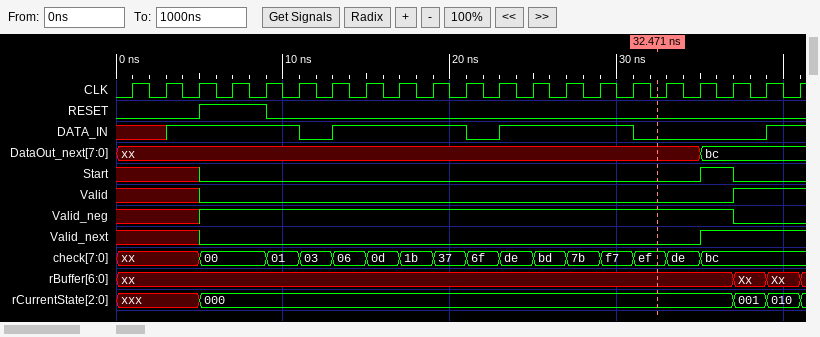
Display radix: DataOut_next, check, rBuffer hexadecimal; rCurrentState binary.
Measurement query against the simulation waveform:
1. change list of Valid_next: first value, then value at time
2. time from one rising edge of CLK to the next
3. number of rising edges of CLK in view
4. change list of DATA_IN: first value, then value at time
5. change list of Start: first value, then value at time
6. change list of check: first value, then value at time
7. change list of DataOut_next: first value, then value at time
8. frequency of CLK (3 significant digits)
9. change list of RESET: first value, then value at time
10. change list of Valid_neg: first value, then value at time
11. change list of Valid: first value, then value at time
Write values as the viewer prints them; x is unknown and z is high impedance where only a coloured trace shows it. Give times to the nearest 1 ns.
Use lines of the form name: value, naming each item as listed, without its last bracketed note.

change list of Valid_next: first value, then value at time: x, 0 at 5 ns, 1 at 35 ns
time from one rising edge of CLK to the next: 2 ns
number of rising edges of CLK in view: 21
change list of DATA_IN: first value, then value at time: x, 1 at 3 ns, 0 at 11 ns, 1 at 13 ns, 0 at 21 ns, 1 at 23 ns, 0 at 31 ns, 1 at 39 ns
change list of Start: first value, then value at time: x, 0 at 5 ns, 1 at 35 ns, 0 at 37 ns
change list of check: first value, then value at time: xx, 00 at 5 ns, 01 at 9 ns, 03 at 11 ns, 06 at 13 ns, 0d at 15 ns, 1b at 17 ns, 37 at 19 ns, 6f at 21 ns, de at 23 ns, bd at 25 ns, 7b at 27 ns, f7 at 29 ns, ef at 31 ns, de at 33 ns, bc at 35 ns
change list of DataOut_next: first value, then value at time: xx, bc at 35 ns
frequency of CLK: 500 MHz
change list of RESET: first value, then value at time: 0, 1 at 5 ns, 0 at 9 ns
change list of Valid_neg: first value, then value at time: x, 1 at 5 ns, 0 at 37 ns
change list of Valid: first value, then value at time: x, 0 at 5 ns, 1 at 37 ns
